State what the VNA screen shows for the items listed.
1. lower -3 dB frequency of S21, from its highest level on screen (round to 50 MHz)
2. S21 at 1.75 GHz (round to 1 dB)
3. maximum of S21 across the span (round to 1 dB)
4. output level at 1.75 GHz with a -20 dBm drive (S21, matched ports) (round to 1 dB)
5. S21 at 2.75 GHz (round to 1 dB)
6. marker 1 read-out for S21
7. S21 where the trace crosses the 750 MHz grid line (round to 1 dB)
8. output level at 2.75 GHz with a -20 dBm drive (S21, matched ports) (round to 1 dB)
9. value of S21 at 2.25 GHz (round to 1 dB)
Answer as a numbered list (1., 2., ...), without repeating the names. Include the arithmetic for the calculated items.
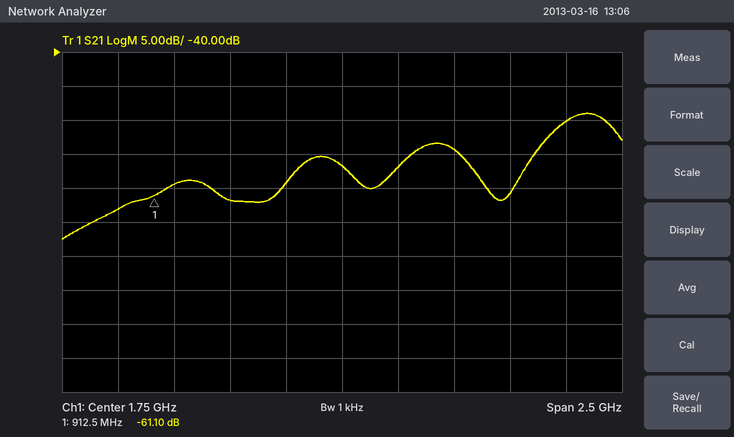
1. 2.70 GHz
2. -57 dB
3. -49 dB
4. -20 dBm + (-57 dB) = -77 dBm
5. -50 dB
6. -61.10 dB
7. -63 dB
8. -20 dBm + (-50 dB) = -70 dBm
9. -54 dB
